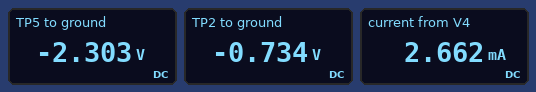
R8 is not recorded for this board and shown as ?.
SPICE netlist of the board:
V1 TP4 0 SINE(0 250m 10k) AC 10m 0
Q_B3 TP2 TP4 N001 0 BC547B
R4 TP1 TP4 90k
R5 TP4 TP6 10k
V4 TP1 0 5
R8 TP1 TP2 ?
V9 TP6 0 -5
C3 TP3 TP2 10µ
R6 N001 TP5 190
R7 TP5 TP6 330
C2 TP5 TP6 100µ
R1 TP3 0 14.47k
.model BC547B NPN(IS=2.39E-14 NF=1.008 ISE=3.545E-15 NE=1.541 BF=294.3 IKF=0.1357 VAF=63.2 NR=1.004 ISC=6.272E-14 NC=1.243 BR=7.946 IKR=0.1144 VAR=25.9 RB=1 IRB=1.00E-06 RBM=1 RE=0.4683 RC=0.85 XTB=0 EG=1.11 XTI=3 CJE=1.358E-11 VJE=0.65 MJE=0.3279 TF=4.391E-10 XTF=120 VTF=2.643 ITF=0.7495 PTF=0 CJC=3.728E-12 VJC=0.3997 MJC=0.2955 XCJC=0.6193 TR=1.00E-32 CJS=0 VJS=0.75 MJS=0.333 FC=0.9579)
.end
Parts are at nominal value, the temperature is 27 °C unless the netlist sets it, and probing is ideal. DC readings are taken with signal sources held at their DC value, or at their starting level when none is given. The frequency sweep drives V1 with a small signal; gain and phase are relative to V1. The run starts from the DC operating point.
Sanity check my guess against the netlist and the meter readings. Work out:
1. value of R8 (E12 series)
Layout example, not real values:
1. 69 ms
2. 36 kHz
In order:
1. 2.2 kΩ
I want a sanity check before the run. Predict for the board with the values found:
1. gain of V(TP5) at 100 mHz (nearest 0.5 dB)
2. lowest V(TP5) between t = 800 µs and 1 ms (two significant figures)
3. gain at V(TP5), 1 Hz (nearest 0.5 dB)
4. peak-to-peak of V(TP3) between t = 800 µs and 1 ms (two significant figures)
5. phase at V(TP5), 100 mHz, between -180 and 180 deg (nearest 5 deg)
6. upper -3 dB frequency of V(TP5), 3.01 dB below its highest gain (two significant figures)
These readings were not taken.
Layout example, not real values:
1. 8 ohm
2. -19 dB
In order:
1. -4.0 dB
2. -2.3 V
3. -4.0 dB
4. 480 mV
5. 0 deg
6. 13 Hz
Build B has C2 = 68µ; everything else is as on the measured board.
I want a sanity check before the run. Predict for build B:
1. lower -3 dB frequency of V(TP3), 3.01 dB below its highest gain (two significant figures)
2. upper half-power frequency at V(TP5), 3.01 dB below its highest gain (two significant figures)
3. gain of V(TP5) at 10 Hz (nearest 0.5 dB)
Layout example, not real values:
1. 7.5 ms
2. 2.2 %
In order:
1. 1.1 Hz
2. 19 Hz
3. -5.0 dB
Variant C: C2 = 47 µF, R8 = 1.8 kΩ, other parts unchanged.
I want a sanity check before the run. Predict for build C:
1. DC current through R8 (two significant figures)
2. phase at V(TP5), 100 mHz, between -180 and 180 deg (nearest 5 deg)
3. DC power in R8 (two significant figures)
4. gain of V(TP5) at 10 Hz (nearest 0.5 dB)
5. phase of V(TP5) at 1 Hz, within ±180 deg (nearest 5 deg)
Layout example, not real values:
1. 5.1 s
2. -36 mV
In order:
1. 3.2 mA
2. 0 deg
3. 18 mW
4. -4.5 dB
5. 0 deg
